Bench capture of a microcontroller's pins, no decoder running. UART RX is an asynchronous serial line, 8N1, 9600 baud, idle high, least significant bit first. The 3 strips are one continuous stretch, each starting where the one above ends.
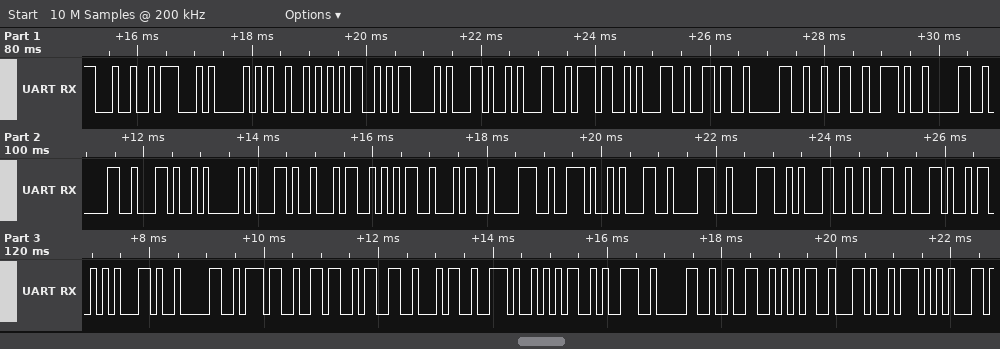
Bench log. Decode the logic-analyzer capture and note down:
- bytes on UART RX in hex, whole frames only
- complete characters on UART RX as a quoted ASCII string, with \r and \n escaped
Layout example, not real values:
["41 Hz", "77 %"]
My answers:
["24 47 50 52 4D 43 2C 31 37 31 36 30 32 2E 30 30 2C 41 2C 34 35 34 38 2E 31 38 38 31 32 2C 53 2C 30 37 36 33 34 2E 35 39 30 32 35 2C 57", "\"$GPRMC,171602.00,A,4548.18812,S,07634.59025,W\""]
